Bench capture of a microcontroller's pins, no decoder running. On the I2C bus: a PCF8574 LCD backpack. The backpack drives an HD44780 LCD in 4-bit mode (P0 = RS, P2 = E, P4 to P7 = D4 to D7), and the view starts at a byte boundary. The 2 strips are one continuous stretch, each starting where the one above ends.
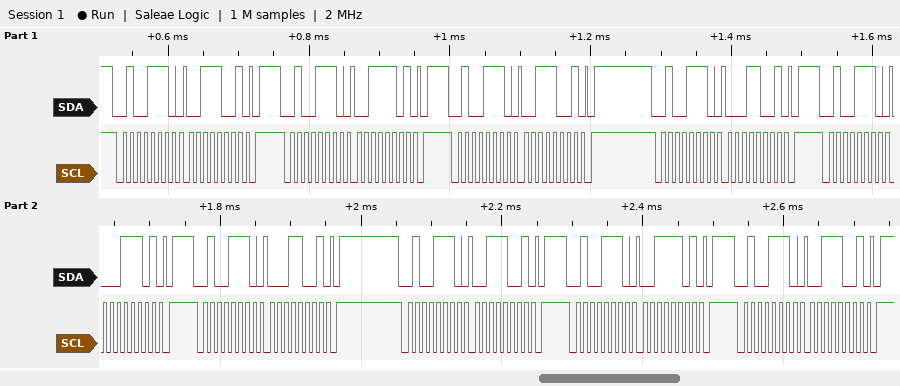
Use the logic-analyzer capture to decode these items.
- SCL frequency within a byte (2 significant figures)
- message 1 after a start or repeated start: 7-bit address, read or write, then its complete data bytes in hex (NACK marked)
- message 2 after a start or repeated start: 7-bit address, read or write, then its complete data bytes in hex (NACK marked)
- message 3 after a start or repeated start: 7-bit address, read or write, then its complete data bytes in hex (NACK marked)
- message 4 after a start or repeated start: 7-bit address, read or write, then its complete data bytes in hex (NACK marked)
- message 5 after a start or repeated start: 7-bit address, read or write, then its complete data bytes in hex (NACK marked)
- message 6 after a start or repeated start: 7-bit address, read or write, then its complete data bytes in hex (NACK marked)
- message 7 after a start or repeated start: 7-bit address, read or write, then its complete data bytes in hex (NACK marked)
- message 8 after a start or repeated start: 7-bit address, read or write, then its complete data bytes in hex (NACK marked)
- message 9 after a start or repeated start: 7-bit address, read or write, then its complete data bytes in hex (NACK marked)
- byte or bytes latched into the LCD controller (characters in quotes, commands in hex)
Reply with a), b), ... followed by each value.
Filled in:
a) 100 kHz
b) 0x27 write: 39
c) 0x27 write: 3D
d) 0x27 write: 39
e) 0x27 write: 19
f) 0x27 write: 1D
g) 0x27 write: 19
h) 0x27 write: 39
i) 0x27 write: 3D
j) 0x27 write: 39
k) '1'
